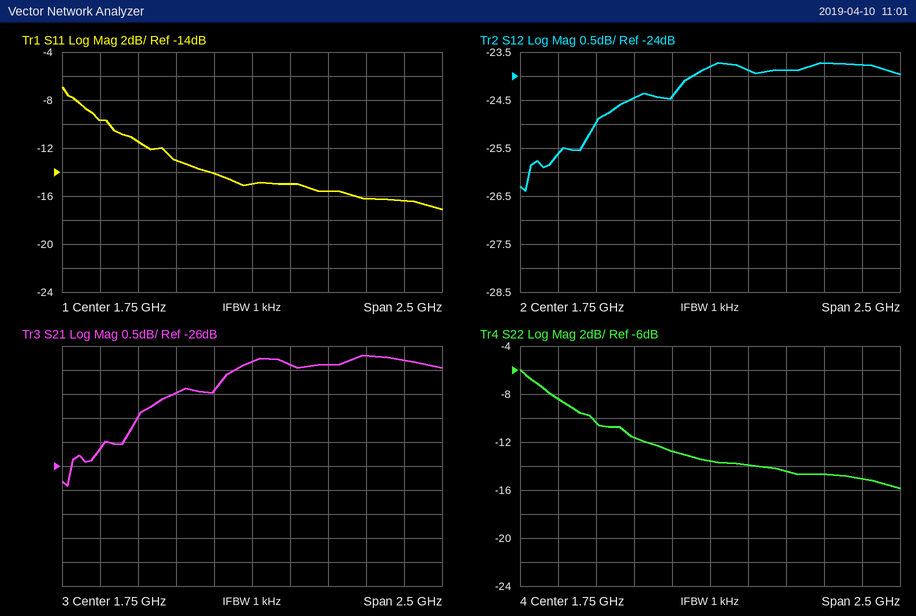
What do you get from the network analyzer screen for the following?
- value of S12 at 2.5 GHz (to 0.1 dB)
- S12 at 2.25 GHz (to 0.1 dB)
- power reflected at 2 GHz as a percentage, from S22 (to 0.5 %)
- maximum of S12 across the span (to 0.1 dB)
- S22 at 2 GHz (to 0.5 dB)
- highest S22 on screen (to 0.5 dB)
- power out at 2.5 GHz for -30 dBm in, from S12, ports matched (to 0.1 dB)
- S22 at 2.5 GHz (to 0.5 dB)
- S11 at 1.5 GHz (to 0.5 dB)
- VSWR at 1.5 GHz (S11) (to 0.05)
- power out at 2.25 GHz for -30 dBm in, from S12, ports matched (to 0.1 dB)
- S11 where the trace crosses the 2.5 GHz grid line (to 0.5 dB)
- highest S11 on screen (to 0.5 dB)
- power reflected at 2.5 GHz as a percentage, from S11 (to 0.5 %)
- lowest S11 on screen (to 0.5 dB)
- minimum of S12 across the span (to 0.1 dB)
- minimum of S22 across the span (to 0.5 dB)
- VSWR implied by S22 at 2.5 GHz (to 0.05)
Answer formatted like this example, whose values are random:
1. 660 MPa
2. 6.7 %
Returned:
1. -23.7 dB
2. -23.9 dB
3. 4.0 %
4. -23.7 dB
5. -14.0 dB
6. -6.0 dB
7. -53.7 dBm
8. -14.5 dB
9. -14.0 dB
10. 1.50
11. -53.9 dBm
12. -16.0 dB
13. -7.0 dB
14. 2.5 %
15. -17.0 dB
16. -26.4 dB
17. -16.0 dB
18. 1.45
